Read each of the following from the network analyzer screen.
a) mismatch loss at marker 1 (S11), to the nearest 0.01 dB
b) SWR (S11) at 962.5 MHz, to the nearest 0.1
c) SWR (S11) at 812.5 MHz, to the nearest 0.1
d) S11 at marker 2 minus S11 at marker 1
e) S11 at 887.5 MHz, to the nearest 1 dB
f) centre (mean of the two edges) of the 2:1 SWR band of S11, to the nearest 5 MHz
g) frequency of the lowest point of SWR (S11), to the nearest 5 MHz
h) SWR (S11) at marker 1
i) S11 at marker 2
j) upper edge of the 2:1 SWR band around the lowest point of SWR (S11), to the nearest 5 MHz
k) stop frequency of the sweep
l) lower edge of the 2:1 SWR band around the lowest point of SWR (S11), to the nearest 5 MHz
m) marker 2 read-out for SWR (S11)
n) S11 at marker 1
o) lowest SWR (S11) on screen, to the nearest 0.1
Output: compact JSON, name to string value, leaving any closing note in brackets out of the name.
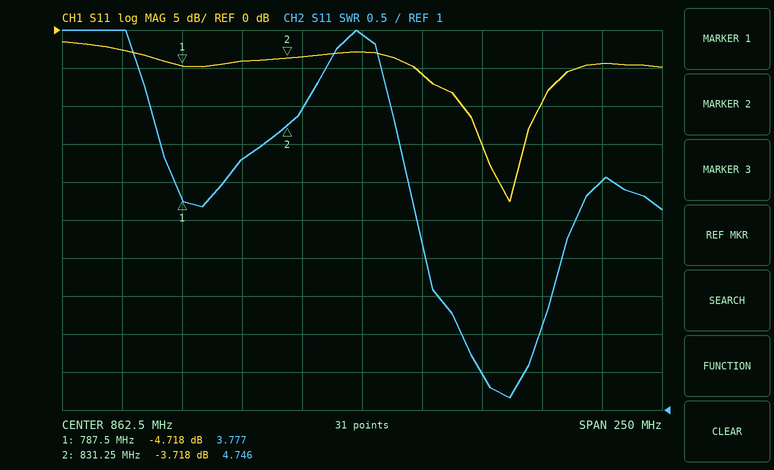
{"mismatch loss at marker 1 (S11), to the nearest 0.01 dB": "1.79 dB", "SWR (S11) at 962.5 MHz, to the nearest 0.1": "4.0", "SWR (S11) at 812.5 MHz, to the nearest 0.1": "4.3", "S11 at marker 2 minus S11 at marker 1": "1.000 dB", "S11 at 887.5 MHz, to the nearest 1 dB": "-6 dB", "centre (mean of the two edges) of the 2:1 SWR band of S11, to the nearest 5 MHz": "920 MHz", "frequency of the lowest point of SWR (S11), to the nearest 5 MHz": "925 MHz", "SWR (S11) at marker 1": "3.777", "S11 at marker 2": "-3.718 dB", "upper edge of the 2:1 SWR band around the lowest point of SWR (S11), to the nearest 5 MHz": "935 MHz", "stop frequency of the sweep": "987.5 MHz", "lower edge of the 2:1 SWR band around the lowest point of SWR (S11), to the nearest 5 MHz": "905 MHz", "marker 2 read-out for SWR": "4.746", "S11 at marker 1": "-4.718 dB", "lowest SWR (S11) on screen, to the nearest 0.1": "1.2"}
